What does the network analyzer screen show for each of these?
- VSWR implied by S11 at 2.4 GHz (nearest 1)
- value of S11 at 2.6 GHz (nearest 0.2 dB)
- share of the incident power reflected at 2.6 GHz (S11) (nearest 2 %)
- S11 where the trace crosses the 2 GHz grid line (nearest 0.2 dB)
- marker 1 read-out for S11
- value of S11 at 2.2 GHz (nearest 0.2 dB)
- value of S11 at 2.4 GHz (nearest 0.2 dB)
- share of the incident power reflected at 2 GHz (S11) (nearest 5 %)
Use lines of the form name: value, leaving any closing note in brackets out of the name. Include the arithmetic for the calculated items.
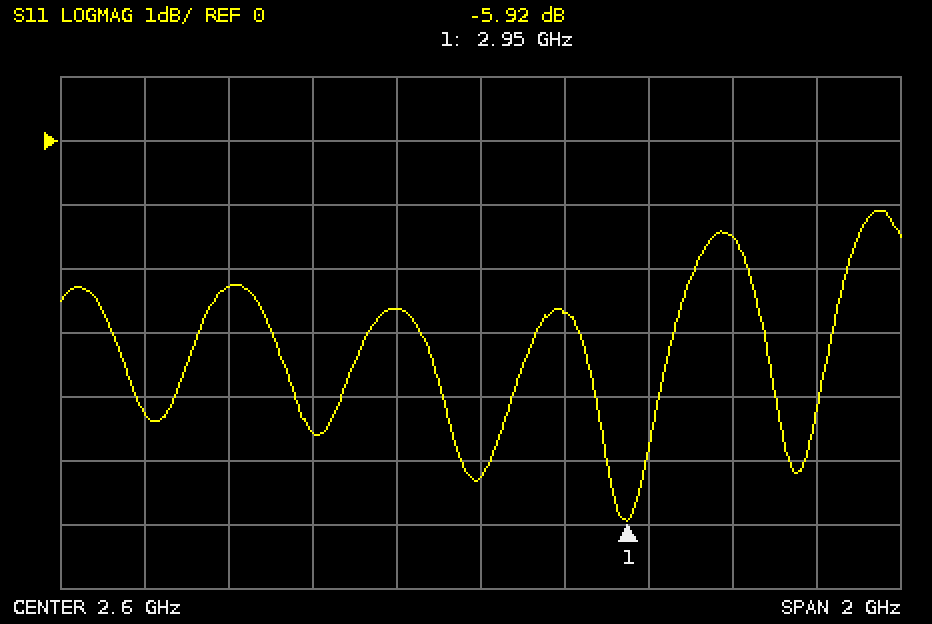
VSWR implied by S11 at 2.4 GHz: |Γ| = 10^(-2.6/20) = 0.7413; VSWR = (1 + 0.7413)/(1 − 0.7413) ≈ 7
value of S11 at 2.6 GHz: -5.2 dB
share of the incident power reflected at 2.6 GHz (S11): 10^(-5.2/10) ≈ 30 %
S11 where the trace crosses the 2 GHz grid line: -2.2 dB
marker 1 read-out for S11: -5.92 dB
value of S11 at 2.2 GHz: -4.6 dB
value of S11 at 2.4 GHz: -2.6 dB
share of the incident power reflected at 2 GHz (S11): 10^(-2.2/10) ≈ 60 %
